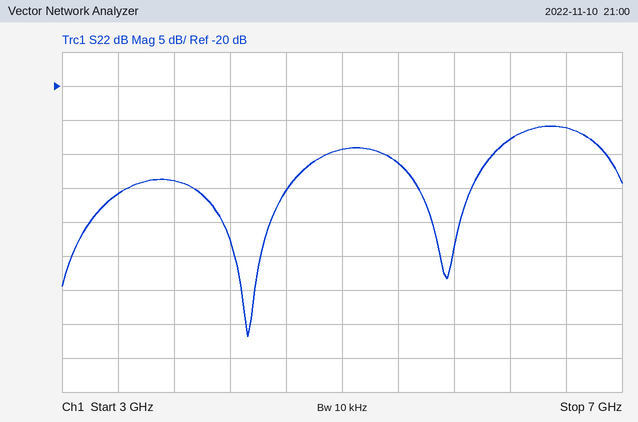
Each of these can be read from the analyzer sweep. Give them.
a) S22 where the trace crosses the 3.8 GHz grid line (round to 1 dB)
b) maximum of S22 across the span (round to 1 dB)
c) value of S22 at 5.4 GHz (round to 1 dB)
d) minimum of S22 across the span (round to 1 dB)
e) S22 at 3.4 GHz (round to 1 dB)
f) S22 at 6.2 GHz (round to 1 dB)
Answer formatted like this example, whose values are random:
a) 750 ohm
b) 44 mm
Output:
a) -34 dB
b) -26 dB
c) -31 dB
d) -57 dB
e) -36 dB
f) -28 dB
